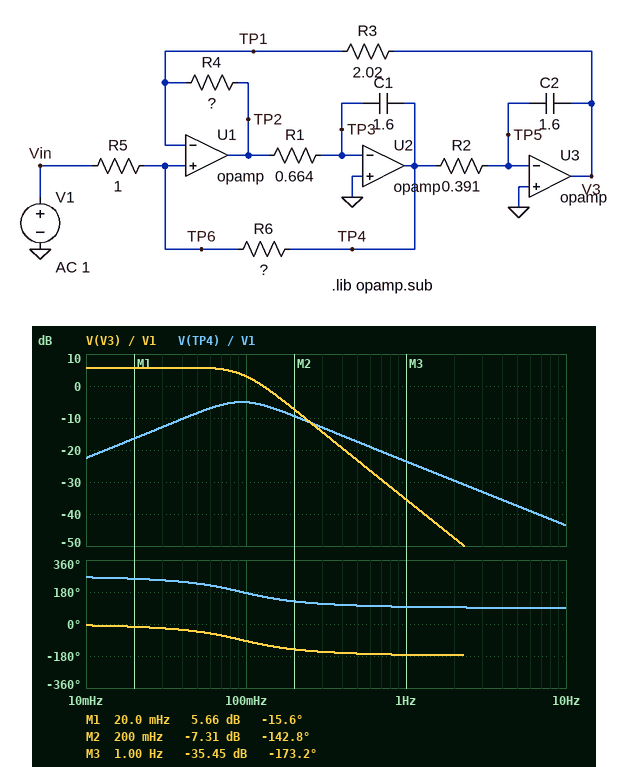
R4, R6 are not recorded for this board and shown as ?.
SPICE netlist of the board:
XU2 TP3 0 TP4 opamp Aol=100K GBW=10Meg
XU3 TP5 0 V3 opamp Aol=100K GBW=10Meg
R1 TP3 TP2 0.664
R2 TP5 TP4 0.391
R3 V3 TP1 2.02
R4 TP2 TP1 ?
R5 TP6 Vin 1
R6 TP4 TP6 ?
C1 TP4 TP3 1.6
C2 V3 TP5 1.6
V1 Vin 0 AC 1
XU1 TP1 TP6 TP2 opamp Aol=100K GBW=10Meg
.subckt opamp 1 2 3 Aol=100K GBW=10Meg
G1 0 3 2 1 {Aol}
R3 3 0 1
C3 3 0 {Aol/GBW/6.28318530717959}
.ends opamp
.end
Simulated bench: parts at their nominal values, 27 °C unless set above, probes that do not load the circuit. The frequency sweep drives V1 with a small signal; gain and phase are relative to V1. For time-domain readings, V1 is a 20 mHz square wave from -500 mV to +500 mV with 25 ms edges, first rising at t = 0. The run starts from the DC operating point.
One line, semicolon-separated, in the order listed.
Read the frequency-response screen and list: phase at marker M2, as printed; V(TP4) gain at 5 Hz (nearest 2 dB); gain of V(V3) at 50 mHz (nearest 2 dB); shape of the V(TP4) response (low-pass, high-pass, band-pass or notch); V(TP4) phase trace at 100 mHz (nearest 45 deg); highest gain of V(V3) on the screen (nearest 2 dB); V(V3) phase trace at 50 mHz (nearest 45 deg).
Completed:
-142.8 deg; -38 dB; 6 dB; band-pass; 180 deg; 6 dB; -45 deg
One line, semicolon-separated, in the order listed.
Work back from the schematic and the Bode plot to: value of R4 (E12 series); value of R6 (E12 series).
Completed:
0.47 Ω; 0.56 Ω
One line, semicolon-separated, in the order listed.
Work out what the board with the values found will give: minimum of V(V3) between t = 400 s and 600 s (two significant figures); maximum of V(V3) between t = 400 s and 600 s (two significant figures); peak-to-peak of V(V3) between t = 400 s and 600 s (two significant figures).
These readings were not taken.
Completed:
-1.1 V; 1.1 V; 2.2 V
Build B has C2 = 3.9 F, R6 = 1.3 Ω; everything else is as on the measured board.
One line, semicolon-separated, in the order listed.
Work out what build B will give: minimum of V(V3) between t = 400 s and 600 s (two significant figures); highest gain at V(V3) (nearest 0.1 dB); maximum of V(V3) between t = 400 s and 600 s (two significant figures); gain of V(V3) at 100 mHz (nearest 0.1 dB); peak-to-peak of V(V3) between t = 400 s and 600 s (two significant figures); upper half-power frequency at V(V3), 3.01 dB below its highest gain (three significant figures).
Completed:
-1.7 V; 9.6 dB; 1.7 V; 0.5 dB; 3.4 V; 63.5 mHz
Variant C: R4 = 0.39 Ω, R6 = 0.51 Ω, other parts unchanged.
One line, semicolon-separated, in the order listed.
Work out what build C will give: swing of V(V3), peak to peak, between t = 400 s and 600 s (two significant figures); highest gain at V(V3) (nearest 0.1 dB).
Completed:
2.3 V; 6.4 dB
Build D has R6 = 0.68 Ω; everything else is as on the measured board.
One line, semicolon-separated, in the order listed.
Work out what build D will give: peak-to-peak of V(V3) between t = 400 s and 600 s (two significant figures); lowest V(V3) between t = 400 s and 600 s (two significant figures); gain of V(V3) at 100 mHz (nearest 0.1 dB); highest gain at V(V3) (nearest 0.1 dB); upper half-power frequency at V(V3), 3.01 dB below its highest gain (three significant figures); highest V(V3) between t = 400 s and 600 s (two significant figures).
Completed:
2.6 V; -1.3 V; 4.7 dB; 7.1 dB; 106 mHz; 1.3 V
